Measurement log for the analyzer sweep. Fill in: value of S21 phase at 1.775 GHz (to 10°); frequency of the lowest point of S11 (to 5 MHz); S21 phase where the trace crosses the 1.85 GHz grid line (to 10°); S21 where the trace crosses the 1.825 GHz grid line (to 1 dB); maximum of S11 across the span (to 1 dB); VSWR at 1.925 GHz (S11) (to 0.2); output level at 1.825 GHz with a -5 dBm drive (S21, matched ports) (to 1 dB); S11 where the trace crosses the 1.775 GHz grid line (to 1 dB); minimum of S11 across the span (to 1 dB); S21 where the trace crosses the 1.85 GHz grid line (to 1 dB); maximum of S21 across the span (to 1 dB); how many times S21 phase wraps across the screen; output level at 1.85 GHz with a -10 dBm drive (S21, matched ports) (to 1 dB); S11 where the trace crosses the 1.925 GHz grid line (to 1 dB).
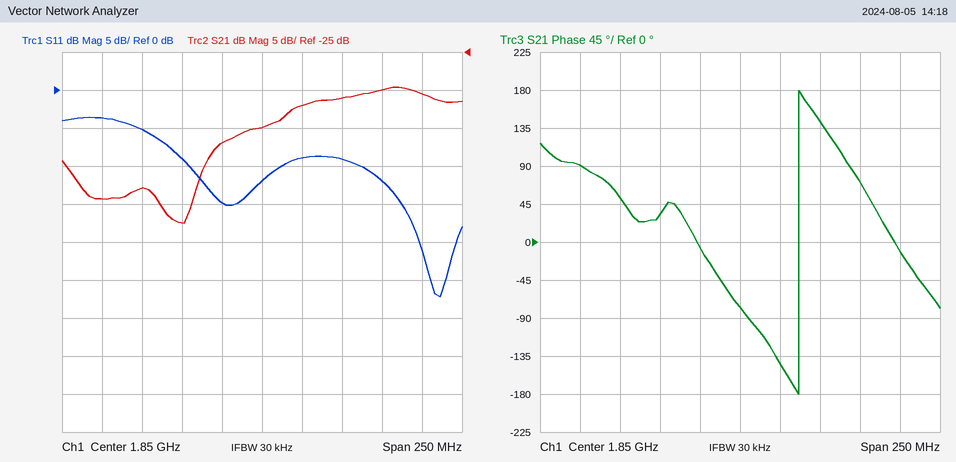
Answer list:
50°
1.960 GHz
-80°
-37 dB
-4 dB
1.6
-42 dBm
-5 dB
-27 dB
-35 dB
-30 dB
1
-45 dBm
-12 dB
